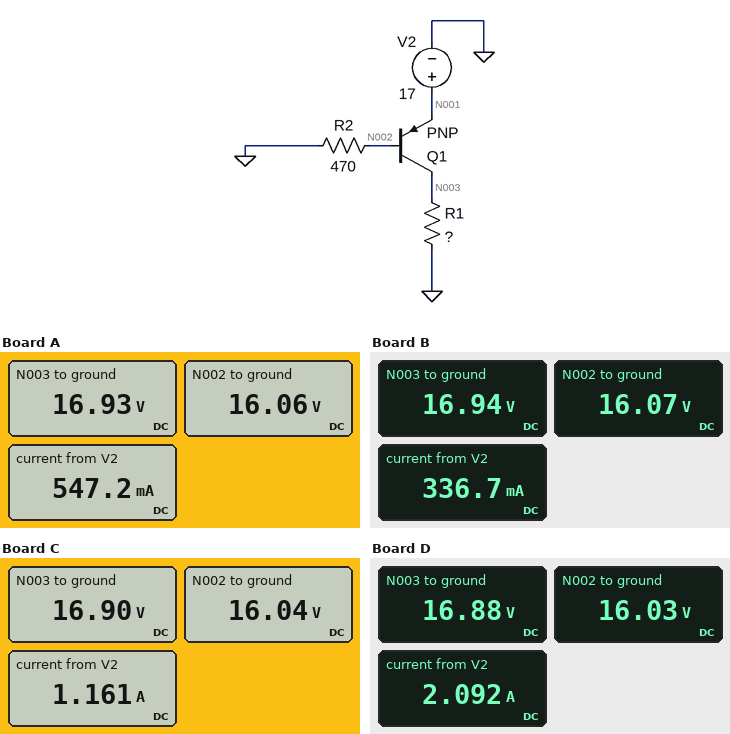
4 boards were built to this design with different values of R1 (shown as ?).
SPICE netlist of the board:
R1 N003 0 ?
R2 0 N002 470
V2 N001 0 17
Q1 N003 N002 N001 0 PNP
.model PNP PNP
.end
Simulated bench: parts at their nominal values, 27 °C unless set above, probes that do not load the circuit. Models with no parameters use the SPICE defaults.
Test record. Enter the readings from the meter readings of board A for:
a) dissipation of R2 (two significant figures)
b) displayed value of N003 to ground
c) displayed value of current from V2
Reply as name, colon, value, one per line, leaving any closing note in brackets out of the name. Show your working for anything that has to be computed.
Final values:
dissipation of R2: (16.06 V)^2 / 470 Ω = 550 mW
displayed value of N003 to ground: 16.93 V
displayed value of current from V2: 547.2 mA
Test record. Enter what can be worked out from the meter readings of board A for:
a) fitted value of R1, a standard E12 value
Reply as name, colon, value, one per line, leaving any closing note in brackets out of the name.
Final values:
fitted value of R1, a standard E12 value: 33 Ω
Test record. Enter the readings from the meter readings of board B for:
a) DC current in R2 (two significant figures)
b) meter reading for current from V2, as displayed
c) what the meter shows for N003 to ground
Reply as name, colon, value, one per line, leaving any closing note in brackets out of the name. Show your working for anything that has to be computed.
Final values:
DC current in R2: (16.07 V) / 470 Ω = 34 mA
meter reading for current from V2, as displayed: 336.7 mA
what the meter shows for N003 to ground: 16.94 V
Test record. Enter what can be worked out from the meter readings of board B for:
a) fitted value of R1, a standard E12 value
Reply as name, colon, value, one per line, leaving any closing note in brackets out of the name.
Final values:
fitted value of R1, a standard E12 value: 56 Ω
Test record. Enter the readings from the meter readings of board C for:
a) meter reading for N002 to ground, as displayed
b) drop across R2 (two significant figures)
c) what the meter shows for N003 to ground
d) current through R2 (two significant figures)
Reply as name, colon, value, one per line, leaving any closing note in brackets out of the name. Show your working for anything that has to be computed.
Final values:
meter reading for N002 to ground, as displayed: 16.04 V
drop across R2: 16.04 V = 16 V
what the meter shows for N003 to ground: 16.90 V
current through R2: (16.04 V) / 470 Ω = 34 mA
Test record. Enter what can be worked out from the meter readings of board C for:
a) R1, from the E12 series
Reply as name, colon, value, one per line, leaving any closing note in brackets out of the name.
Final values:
R1, from the E12 series: 15 Ω
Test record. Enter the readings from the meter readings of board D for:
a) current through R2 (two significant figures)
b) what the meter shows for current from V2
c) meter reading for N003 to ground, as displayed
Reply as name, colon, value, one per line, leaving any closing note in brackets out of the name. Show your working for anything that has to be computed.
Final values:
current through R2: (16.03 V) / 470 Ω = 34 mA
what the meter shows for current from V2: 2.092 A
meter reading for N003 to ground, as displayed: 16.88 V
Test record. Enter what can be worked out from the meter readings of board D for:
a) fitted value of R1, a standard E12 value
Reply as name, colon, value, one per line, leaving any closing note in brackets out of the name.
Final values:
fitted value of R1, a standard E12 value: 8.2 Ω
